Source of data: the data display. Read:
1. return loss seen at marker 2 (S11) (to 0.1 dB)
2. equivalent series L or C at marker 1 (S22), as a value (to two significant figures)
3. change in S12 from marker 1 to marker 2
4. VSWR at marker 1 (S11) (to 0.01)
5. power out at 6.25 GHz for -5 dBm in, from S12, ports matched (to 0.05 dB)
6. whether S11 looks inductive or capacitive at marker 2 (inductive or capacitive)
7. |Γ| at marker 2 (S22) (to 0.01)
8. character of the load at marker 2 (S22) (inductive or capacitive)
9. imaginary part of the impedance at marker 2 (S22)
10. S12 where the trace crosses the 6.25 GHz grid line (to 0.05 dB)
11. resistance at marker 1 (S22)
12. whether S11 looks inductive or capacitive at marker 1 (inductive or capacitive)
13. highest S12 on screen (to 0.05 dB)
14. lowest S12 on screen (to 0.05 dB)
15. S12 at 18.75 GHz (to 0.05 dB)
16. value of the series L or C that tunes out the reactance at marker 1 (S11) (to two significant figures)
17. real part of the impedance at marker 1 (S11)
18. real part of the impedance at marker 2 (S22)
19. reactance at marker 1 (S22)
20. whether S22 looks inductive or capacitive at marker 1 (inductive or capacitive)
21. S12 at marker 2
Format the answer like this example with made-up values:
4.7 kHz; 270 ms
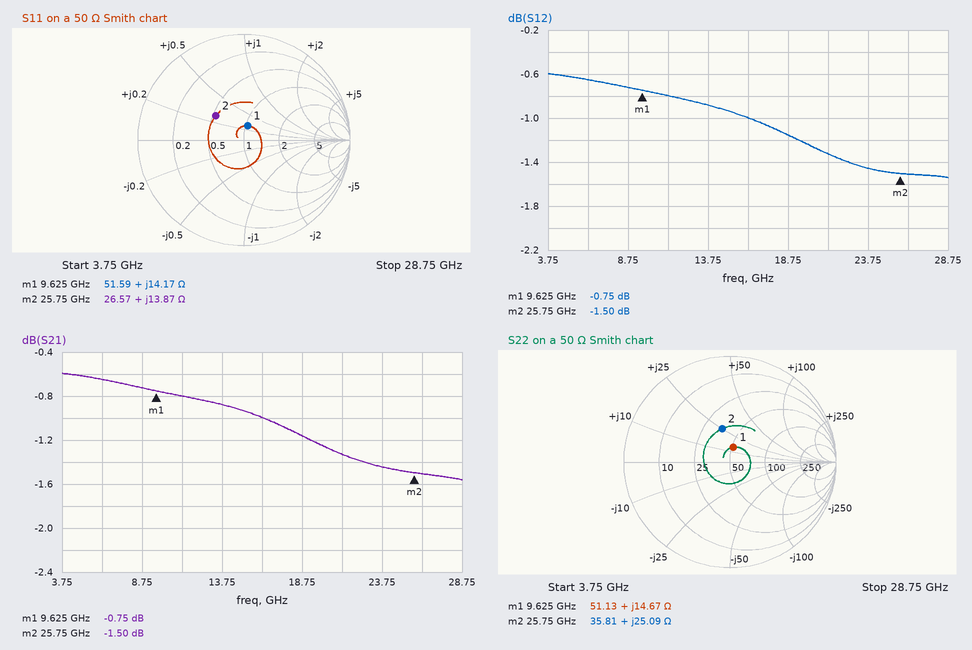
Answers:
9.1 dB; 240 pH; -0.75 dB; 1.32; -5.65 dBm; inductive; 0.32; inductive; +25.09 Ω; -0.65 dB; 51.13 Ω; inductive; -0.60 dB; -1.55 dB; -1.15 dB; 1.2 pF; 51.59 Ω; 35.81 Ω; +14.67 Ω; inductive; -1.50 dB
